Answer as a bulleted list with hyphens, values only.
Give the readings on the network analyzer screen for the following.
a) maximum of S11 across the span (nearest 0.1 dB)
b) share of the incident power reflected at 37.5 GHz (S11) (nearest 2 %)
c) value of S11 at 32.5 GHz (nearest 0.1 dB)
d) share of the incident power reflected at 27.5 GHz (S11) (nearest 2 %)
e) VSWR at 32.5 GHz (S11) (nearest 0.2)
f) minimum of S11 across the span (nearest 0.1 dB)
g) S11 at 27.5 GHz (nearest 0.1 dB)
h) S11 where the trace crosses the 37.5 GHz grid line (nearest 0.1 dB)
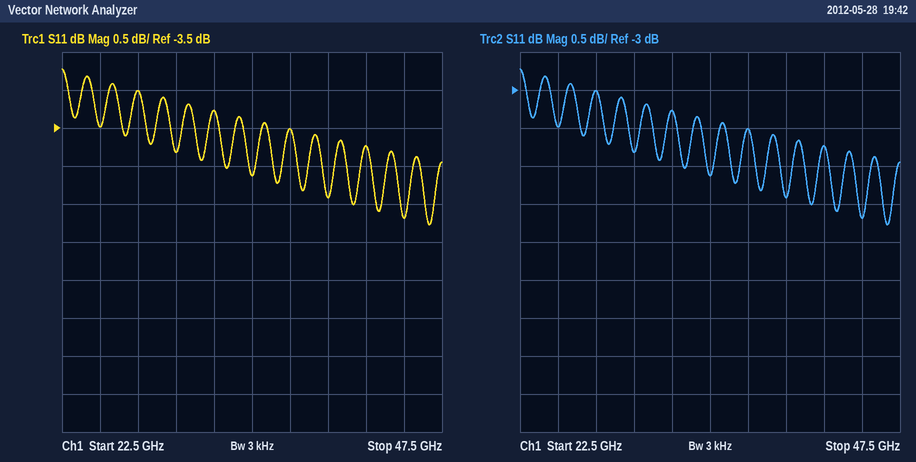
- -2.7 dB
- 44 %
- -3.3 dB
- 50 %
- 5.4
- -4.8 dB
- -3.0 dB
- -3.5 dB
